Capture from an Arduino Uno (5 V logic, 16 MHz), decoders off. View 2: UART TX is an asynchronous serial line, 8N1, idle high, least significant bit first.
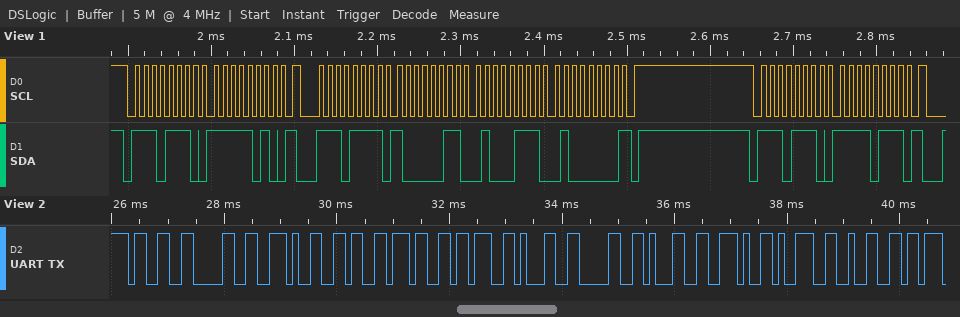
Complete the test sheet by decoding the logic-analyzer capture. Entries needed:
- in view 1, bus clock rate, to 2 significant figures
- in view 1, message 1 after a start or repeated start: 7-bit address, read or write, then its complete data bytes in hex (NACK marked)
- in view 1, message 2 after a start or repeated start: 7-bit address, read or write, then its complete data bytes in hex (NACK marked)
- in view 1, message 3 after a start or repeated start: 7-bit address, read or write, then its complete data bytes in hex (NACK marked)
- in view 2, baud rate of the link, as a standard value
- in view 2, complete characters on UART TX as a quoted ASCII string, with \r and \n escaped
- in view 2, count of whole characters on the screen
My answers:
100 kHz
0x77 write: FA
0x77 read: 83 47 40 NACK
0x77 write: F7
9600 baud
"30.67;101.92"
12
